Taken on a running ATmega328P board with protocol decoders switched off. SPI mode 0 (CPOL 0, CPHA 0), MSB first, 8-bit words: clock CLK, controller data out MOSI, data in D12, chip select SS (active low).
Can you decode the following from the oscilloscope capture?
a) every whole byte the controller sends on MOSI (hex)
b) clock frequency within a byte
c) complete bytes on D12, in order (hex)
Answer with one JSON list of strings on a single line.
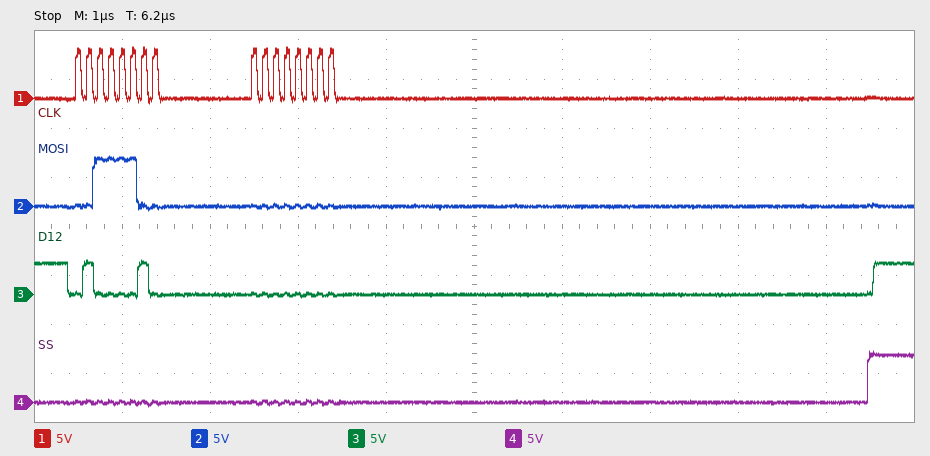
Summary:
["0x3C 0x00", "8 MHz", "0x42 0x00"]
